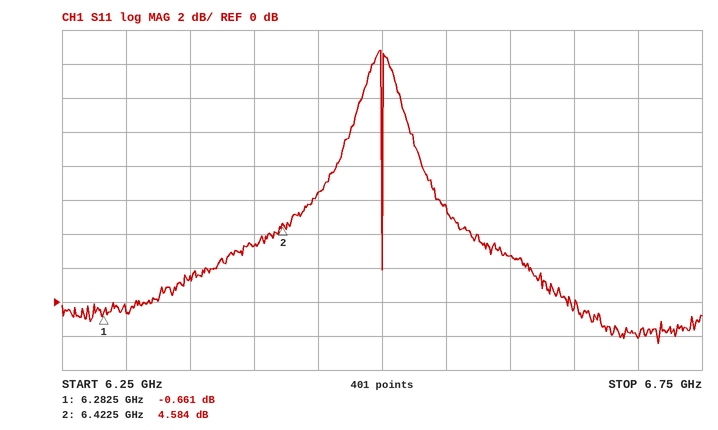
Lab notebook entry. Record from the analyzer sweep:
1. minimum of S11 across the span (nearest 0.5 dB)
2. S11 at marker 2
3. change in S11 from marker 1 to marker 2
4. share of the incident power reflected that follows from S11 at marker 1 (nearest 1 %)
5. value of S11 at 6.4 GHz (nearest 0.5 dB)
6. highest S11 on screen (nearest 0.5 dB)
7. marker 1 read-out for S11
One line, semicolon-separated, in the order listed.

-2.5 dB; 4.584 dB; 5.245 dB; 86 %; 3.5 dB; 15.0 dB; -0.661 dB
